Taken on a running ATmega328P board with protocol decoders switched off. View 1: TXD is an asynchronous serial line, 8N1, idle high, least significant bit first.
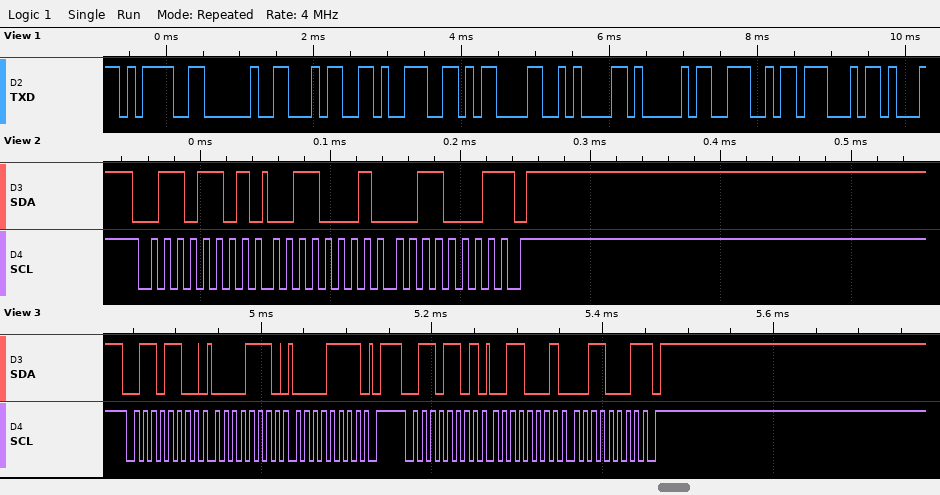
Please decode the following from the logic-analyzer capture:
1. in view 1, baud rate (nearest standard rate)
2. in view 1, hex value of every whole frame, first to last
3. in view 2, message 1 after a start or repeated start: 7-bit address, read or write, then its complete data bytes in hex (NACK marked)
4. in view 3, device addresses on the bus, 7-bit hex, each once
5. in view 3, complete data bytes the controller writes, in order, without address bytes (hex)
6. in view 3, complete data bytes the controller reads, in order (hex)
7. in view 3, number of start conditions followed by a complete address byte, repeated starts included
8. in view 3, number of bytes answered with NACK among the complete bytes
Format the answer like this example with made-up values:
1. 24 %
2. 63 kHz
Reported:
1. 9600 baud
2. 3D 20 34 39 0D 0A 41 4E 47
3. 0x36 read: 31 31 NACK
4. 0x36
5. 0E 0F
6. 31 31
7. 2
8. 1
